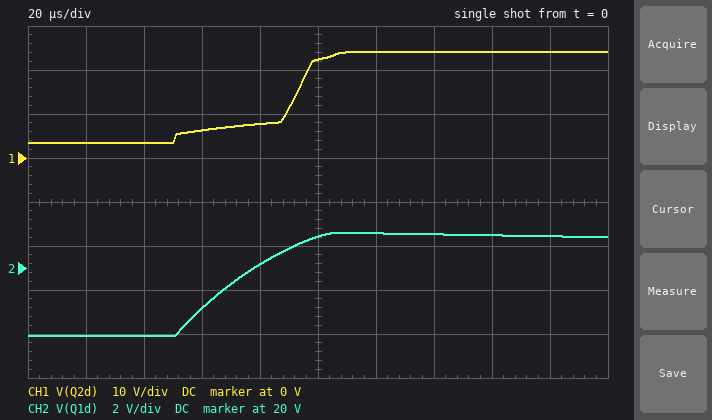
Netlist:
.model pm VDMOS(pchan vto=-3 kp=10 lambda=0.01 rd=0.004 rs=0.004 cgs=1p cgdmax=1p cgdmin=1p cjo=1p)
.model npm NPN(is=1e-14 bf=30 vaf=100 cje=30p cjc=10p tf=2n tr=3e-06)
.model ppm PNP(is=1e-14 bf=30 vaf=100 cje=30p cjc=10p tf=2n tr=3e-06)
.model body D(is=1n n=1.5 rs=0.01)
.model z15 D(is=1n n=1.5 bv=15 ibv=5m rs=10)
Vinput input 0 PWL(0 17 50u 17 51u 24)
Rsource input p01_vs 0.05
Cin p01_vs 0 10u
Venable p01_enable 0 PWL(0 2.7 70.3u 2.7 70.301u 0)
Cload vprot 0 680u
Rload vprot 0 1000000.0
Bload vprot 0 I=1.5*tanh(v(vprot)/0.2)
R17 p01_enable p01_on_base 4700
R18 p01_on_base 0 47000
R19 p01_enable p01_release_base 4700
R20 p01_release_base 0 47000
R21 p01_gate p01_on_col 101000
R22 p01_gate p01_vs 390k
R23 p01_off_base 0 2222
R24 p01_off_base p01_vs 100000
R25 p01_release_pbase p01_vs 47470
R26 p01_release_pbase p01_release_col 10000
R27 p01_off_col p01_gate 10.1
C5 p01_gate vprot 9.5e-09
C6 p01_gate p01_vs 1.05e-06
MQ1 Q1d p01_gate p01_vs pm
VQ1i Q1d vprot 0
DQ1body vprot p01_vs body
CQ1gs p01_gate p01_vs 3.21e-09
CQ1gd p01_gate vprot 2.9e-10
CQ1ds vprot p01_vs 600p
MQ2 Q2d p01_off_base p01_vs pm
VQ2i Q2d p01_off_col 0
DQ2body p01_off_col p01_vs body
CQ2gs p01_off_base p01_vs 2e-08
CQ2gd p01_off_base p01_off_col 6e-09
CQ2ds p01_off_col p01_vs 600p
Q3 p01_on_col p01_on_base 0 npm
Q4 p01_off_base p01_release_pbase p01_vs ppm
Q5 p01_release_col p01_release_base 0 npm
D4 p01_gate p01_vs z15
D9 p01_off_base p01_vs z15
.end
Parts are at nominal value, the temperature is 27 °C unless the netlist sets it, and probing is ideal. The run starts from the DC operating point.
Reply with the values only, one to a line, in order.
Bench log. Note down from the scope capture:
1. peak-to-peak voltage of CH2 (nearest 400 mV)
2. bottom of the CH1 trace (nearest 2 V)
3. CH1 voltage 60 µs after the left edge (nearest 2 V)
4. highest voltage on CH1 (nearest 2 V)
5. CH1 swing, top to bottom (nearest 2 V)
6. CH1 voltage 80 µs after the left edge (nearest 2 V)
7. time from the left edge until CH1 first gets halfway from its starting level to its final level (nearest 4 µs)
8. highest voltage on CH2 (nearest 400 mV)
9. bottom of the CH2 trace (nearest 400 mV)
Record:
4.8 V
4 V
6 V
24 V
20 V
8 V
92 µs
21.6 V
16.8 V
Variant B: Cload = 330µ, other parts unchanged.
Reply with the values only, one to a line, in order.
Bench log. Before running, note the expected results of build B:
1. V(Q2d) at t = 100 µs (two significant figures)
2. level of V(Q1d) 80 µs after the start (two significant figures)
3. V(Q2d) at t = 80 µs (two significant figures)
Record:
23 V
22 V
9.0 V
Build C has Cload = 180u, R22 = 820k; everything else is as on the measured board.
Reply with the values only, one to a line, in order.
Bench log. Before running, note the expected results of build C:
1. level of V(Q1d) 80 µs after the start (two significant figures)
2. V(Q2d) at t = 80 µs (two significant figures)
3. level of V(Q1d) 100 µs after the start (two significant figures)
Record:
23 V
8.7 V
24 V
